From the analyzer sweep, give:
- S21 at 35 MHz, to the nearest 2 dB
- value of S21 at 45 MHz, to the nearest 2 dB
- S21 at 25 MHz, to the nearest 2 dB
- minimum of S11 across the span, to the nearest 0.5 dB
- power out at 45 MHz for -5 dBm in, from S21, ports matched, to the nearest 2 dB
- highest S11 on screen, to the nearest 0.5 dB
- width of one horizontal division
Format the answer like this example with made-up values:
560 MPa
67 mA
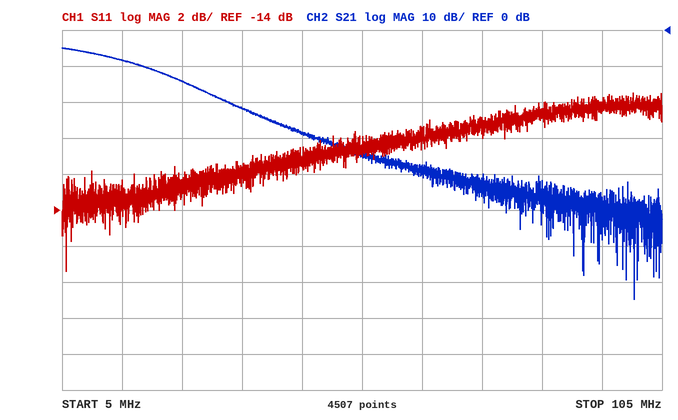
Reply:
-22 dB
-28 dB
-14 dB
-17.5 dB
-34 dBm
-7.5 dB
10 MHz
